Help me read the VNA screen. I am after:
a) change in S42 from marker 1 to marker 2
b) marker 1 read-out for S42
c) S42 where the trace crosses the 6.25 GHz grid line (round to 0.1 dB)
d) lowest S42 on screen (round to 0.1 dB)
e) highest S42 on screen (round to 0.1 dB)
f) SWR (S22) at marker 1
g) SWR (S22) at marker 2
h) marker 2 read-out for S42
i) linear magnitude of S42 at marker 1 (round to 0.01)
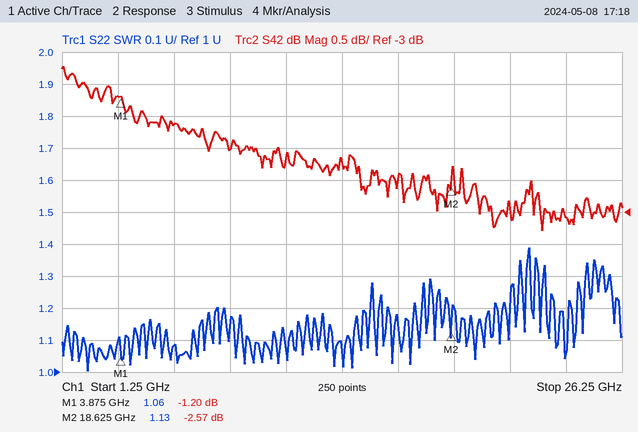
-1.37 dB
-1.20 dB
-1.6 dB
-3.3 dB
-0.7 dB
1.06
1.13
-2.57 dB
0.87
